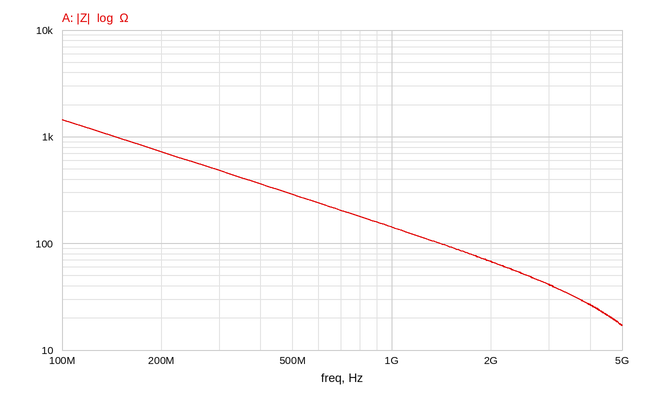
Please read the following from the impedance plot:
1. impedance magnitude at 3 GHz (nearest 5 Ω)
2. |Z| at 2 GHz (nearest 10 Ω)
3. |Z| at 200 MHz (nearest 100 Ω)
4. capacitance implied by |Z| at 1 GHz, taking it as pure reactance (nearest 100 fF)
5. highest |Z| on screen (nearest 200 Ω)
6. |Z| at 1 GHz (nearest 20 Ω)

40 Ω
70 Ω
700 Ω
1.1 pF
1.4 kΩ
140 Ω
